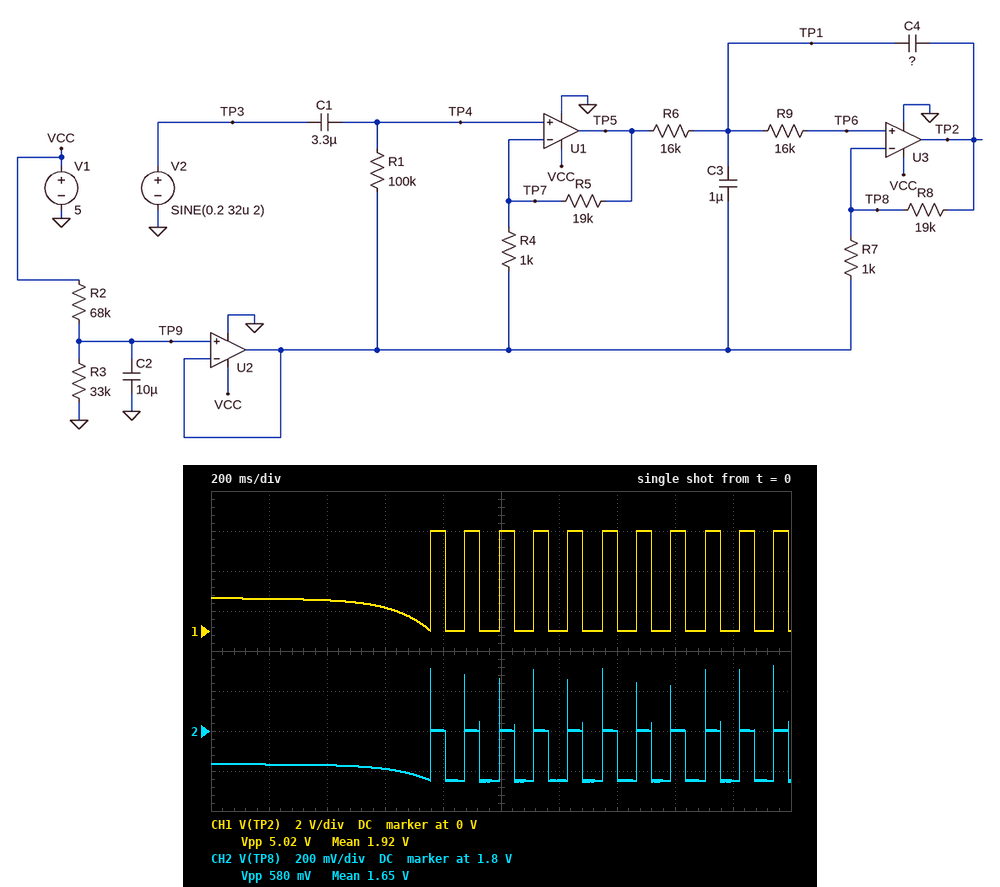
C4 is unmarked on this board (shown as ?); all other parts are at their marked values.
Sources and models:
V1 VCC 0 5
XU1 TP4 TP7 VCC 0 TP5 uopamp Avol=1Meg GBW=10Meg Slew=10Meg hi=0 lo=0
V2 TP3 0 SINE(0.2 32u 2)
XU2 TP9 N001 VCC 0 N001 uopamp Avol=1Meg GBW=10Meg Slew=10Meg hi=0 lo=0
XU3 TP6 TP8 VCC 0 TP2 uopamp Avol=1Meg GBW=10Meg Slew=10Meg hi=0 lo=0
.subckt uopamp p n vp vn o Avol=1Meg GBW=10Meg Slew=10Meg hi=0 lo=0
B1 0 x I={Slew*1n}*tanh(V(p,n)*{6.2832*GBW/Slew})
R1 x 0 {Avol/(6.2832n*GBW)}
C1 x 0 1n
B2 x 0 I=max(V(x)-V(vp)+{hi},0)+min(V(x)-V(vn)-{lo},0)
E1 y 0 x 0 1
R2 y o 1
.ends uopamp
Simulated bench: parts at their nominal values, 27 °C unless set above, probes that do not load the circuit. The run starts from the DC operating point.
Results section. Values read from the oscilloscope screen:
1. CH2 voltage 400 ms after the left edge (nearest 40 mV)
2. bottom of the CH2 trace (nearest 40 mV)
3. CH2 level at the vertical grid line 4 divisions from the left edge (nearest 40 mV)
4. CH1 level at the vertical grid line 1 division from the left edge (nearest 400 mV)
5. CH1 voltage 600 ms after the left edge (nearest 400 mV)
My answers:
1.64 V
1.56 V
1.80 V
1.6 V
1.2 V
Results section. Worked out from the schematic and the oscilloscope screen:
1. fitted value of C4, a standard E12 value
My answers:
470 nF
